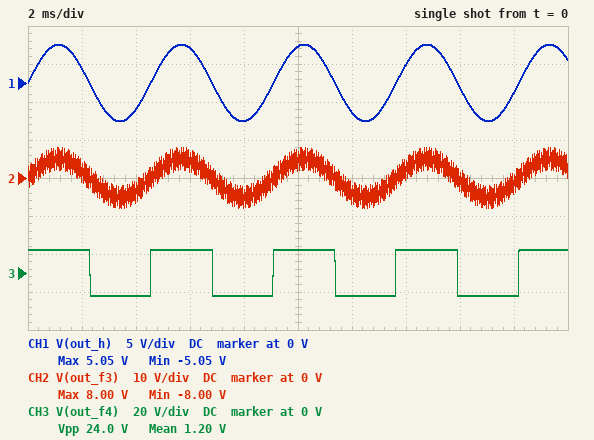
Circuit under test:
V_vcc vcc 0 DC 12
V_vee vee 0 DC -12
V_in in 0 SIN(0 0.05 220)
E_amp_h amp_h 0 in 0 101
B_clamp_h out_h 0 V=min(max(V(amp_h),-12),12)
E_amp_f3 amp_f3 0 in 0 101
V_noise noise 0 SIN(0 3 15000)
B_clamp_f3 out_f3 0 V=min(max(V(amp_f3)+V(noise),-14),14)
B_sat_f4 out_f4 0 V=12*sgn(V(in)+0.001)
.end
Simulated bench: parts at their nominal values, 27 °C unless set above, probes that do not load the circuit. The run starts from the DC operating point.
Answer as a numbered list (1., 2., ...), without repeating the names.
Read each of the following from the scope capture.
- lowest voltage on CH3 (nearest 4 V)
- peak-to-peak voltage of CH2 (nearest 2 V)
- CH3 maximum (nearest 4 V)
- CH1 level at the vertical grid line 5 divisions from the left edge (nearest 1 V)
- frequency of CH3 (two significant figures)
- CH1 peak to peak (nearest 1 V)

1. -12 V
2. 16 V
3. 12 V
4. 5 V
5. 220 Hz
6. 10 V
